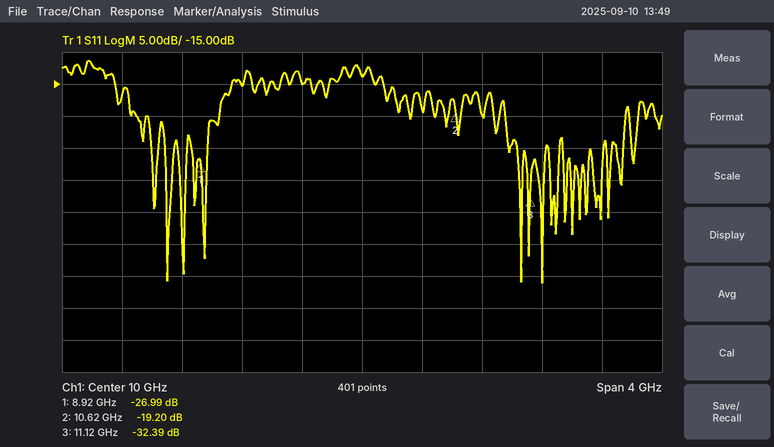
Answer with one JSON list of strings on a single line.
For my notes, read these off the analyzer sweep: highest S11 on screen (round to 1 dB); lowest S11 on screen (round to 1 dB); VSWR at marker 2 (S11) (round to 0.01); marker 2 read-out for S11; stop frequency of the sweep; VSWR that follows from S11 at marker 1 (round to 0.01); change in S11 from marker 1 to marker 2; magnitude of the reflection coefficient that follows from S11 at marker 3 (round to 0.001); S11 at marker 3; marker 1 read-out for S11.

["-11 dB", "-46 dB", "1.25", "-19.20 dB", "12 GHz", "1.09", "7.79 dB", "0.024", "-32.39 dB", "-26.99 dB"]
